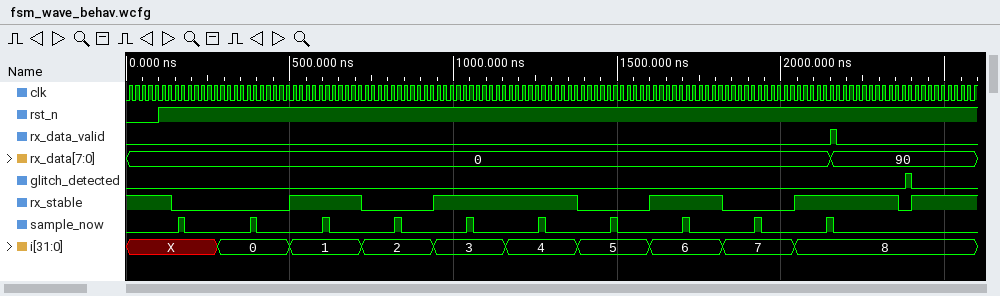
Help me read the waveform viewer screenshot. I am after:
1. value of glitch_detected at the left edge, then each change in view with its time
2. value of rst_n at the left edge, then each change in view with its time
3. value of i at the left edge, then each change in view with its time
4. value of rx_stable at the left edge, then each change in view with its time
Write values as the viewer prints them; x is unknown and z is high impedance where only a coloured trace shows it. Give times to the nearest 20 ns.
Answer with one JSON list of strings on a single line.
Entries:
["0, 1 at 2380 ns, 0 at 2400 ns", "0, 1 at 100 ns", "X, 0 at 280 ns, 1 at 500 ns, 2 at 720 ns, 3 at 940 ns, 4 at 1160 ns, 5 at 1380 ns, 6 at 1600 ns, 7 at 1820 ns, 8 at 2040 ns", "1, 0 at 140 ns, 1 at 500 ns, 0 at 720 ns, 1 at 940 ns, 0 at 1380 ns, 1 at 1600 ns, 0 at 1820 ns, 1 at 2040 ns, 0 at 2360 ns, 1 at 2400 ns"]
